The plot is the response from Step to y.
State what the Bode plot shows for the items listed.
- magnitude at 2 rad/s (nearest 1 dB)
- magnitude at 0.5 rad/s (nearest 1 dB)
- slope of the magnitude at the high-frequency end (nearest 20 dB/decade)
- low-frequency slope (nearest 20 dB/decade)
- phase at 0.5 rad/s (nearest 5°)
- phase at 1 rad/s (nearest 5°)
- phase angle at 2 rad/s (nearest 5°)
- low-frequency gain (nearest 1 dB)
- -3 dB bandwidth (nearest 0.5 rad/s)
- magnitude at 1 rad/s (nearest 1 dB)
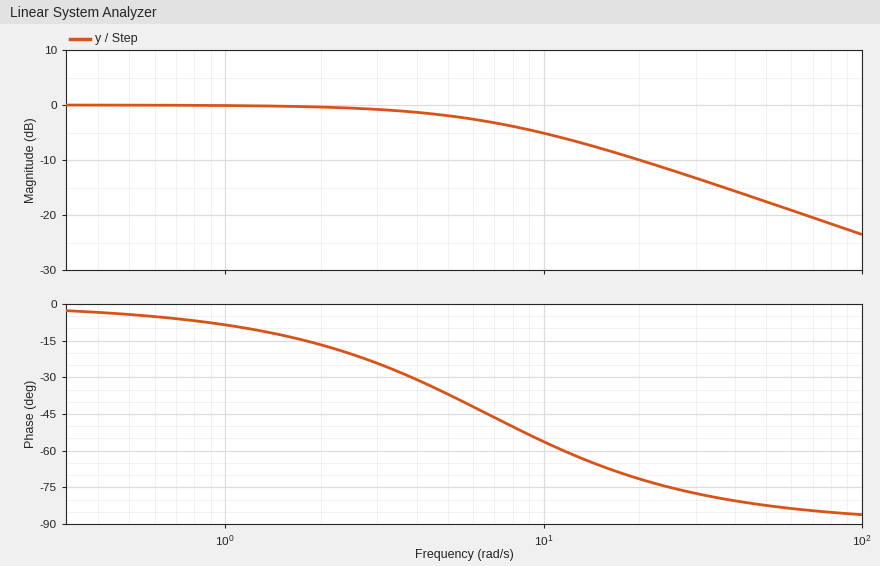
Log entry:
0 dB
0 dB
-20 dB/decade
0 dB/decade
-5°
-10°
-15°
0 dB
6.5 rad/s
0 dB
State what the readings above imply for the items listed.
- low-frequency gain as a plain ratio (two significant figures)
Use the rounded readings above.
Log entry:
1.0
